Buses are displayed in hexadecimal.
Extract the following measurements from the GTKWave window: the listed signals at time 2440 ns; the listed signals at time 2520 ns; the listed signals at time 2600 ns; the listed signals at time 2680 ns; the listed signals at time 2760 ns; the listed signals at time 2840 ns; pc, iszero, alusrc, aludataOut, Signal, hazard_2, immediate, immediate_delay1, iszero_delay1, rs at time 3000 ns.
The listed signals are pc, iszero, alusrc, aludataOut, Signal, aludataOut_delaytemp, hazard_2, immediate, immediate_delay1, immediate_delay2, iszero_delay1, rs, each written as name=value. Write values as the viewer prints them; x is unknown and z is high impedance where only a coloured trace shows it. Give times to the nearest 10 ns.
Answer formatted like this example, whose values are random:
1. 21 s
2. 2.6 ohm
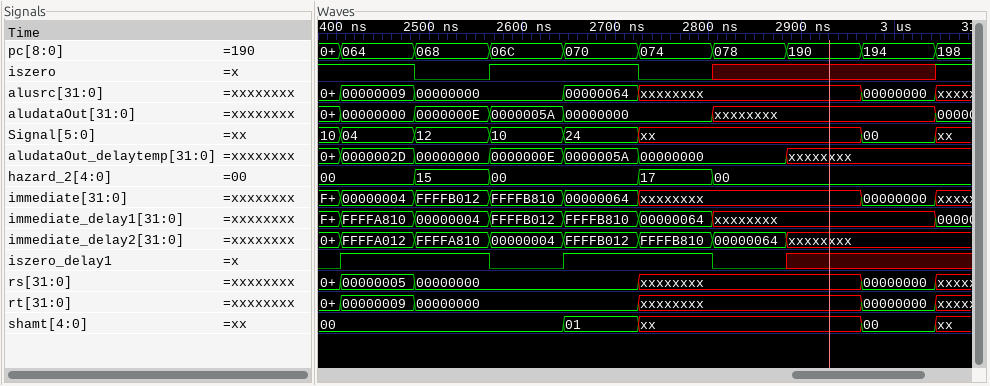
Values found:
1. pc=064, iszero=1, alusrc=00000009, aludataOut=00000000, Signal=04, aludataOut_delaytemp=0000002D, hazard_2=00, immediate=00000004, immediate_delay1=FFFFA810, immediate_delay2=FFFFA012, iszero_delay1=1, rs=00000005
2. pc=068, iszero=0, alusrc=00000000, aludataOut=0000000E, Signal=12, aludataOut_delaytemp=00000000, hazard_2=15, immediate=FFFFB012, immediate_delay1=00000004, immediate_delay2=FFFFA810, iszero_delay1=1, rs=00000000
3. pc=06C, iszero=1, alusrc=00000000, aludataOut=0000005A, Signal=10, aludataOut_delaytemp=0000000E, hazard_2=00, immediate=FFFFB810, immediate_delay1=FFFFB012, immediate_delay2=00000004, iszero_delay1=0, rs=00000000
4. pc=070, iszero=1, alusrc=00000064, aludataOut=00000000, Signal=24, aludataOut_delaytemp=0000005A, hazard_2=00, immediate=00000064, immediate_delay1=FFFFB810, immediate_delay2=FFFFB012, iszero_delay1=1, rs=00000000
5. pc=074, iszero=0, alusrc=xxxxxxxx, aludataOut=00000000, Signal=xx, aludataOut_delaytemp=00000000, hazard_2=17, immediate=xxxxxxxx, immediate_delay1=00000064, immediate_delay2=FFFFB810, iszero_delay1=1, rs=xxxxxxxx
6. pc=078, iszero=x, alusrc=xxxxxxxx, aludataOut=xxxxxxxx, Signal=xx, aludataOut_delaytemp=00000000, hazard_2=00, immediate=xxxxxxxx, immediate_delay1=xxxxxxxx, immediate_delay2=00000064, iszero_delay1=0, rs=xxxxxxxx
7. pc=194, iszero=x, alusrc=00000000, aludataOut=xxxxxxxx, Signal=00, hazard_2=00, immediate=00000000, immediate_delay1=xxxxxxxx, iszero_delay1=x, rs=00000000
